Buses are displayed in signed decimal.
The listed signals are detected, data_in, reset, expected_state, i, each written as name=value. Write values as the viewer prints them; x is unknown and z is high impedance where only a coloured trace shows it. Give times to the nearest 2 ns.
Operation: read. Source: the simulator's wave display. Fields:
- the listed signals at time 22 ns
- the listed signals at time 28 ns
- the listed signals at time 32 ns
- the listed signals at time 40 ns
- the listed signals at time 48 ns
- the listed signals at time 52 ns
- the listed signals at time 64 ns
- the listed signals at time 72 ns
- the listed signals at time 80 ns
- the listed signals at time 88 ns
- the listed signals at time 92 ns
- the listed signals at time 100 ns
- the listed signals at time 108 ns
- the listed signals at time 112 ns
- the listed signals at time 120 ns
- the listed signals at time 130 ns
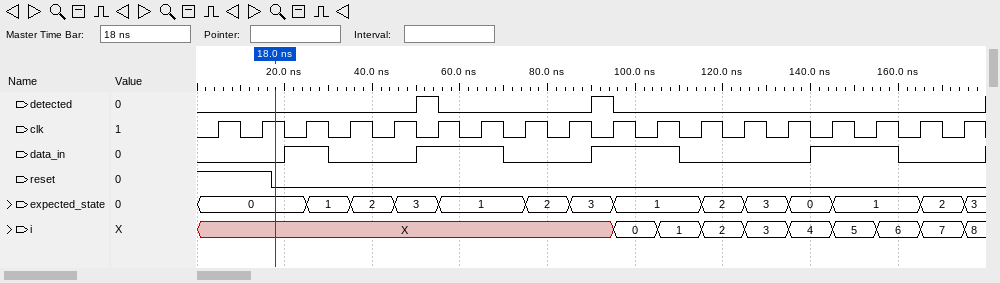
detected=0, data_in=1, reset=0, expected_state=0, i=X
detected=0, data_in=1, reset=0, expected_state=1, i=X
detected=0, data_in=0, reset=0, expected_state=1, i=X
detected=0, data_in=0, reset=0, expected_state=2, i=X
detected=0, data_in=0, reset=0, expected_state=3, i=X
detected=1, data_in=1, reset=0, expected_state=3, i=X
detected=0, data_in=1, reset=0, expected_state=1, i=X
detected=0, data_in=0, reset=0, expected_state=1, i=X
detected=0, data_in=0, reset=0, expected_state=2, i=X
detected=0, data_in=0, reset=0, expected_state=3, i=X
detected=1, data_in=1, reset=0, expected_state=3, i=X
detected=0, data_in=1, reset=0, expected_state=1, i=0
detected=0, data_in=1, reset=0, expected_state=1, i=1
detected=0, data_in=0, reset=0, expected_state=1, i=1
detected=0, data_in=0, reset=0, expected_state=2, i=2
detected=0, data_in=0, reset=0, expected_state=3, i=3
